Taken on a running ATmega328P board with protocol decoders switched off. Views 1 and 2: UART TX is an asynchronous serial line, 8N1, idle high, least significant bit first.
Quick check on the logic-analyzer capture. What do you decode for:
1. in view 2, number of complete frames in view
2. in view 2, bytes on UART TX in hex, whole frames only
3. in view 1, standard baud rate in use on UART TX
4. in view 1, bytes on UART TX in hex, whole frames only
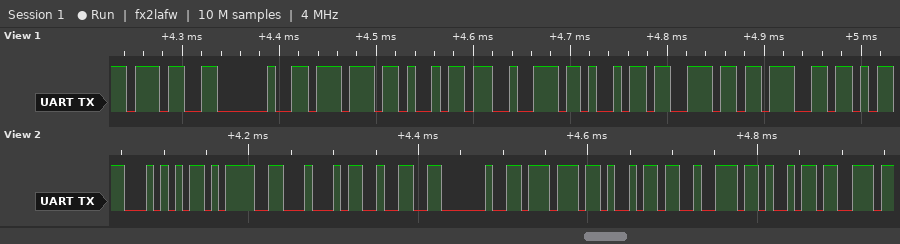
9
54 3D 44 32 20 77 69 72 69
115200 baud
0x37 0x20 0x77 0x69 0x72 0x69 0x6E 0x67
